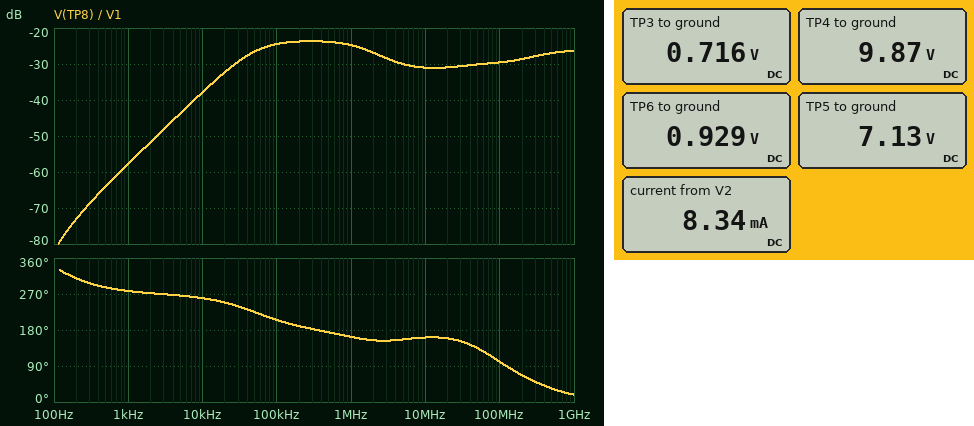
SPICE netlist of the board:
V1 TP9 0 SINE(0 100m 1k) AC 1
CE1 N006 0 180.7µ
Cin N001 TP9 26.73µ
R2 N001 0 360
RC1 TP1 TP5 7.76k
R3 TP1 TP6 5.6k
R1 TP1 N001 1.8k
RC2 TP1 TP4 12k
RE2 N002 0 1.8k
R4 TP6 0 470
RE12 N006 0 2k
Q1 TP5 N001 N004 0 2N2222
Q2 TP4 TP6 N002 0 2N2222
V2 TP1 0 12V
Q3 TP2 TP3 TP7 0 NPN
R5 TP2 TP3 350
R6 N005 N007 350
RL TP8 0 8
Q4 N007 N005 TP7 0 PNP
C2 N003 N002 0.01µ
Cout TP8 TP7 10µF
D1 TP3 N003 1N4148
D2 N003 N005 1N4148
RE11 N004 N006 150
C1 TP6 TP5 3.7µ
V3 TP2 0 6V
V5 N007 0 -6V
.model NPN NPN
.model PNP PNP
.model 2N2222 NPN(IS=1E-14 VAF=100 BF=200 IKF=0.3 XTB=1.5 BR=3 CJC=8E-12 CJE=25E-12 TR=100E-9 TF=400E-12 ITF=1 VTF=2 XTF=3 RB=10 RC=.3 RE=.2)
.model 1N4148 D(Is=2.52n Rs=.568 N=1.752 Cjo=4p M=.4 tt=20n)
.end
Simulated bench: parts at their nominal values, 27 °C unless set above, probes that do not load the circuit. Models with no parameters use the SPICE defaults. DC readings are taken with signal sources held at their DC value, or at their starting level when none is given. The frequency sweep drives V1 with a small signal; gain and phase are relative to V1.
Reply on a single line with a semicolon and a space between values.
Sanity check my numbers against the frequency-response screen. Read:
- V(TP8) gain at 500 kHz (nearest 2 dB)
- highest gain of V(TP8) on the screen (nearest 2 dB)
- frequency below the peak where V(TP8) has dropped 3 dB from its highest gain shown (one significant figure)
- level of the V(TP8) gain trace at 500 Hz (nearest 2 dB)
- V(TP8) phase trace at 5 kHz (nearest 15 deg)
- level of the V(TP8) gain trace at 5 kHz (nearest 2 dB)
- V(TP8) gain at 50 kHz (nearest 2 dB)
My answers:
-24 dB; -24 dB; 50 kHz; -64 dB; 270 deg; -44 dB; -26 dB
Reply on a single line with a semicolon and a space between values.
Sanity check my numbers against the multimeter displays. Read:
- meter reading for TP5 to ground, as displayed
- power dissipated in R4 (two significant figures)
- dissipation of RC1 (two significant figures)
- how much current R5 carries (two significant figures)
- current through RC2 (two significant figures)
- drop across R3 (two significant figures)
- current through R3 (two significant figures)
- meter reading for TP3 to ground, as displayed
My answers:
7.13 V; 1.8 mW; 3.1 mW; 15 mA; 180 µA; 11 V; 2.0 mA; 0.716 V
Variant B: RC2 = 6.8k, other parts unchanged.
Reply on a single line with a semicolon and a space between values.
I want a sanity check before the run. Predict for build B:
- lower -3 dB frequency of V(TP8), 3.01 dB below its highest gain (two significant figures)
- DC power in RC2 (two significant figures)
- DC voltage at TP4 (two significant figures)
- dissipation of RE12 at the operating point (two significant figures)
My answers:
50 kHz; 210 µW; 11 V; 800 µW
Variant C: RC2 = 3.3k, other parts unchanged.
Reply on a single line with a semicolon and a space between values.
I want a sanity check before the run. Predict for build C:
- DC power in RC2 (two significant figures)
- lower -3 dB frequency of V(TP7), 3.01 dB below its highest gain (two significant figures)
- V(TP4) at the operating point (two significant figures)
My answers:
100 µW; 50 kHz; 11 V
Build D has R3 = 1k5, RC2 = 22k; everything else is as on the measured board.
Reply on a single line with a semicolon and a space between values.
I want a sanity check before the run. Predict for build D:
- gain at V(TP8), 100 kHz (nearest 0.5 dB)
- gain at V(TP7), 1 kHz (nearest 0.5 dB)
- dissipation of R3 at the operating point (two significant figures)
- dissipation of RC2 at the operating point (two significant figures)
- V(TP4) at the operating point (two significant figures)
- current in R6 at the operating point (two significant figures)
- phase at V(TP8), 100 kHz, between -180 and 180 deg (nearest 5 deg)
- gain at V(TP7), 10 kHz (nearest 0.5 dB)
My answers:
-30.5 dB; -53.5 dB; 58 mW; 4.6 mW; 2.0 V; 15 mA; -160 deg; -40.5 dB
